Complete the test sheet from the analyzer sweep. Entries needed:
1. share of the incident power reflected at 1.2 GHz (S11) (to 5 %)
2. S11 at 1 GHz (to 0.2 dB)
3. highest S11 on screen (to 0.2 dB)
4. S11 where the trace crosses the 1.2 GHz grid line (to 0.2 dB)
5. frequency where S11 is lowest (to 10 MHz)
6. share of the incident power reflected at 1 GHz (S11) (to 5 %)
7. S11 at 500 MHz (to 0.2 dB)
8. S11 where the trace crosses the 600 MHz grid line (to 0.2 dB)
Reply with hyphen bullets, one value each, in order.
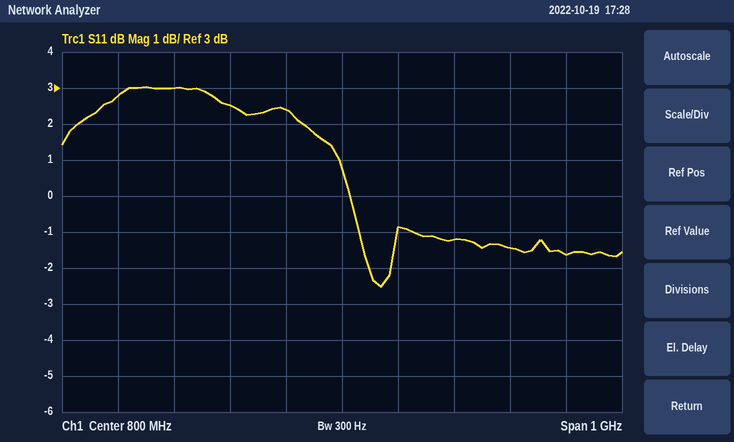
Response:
- 70 %
- -1.2 dB
- 3.0 dB
- -1.6 dB
- 870 MHz
- 75 %
- 3.0 dB
- 2.6 dB
